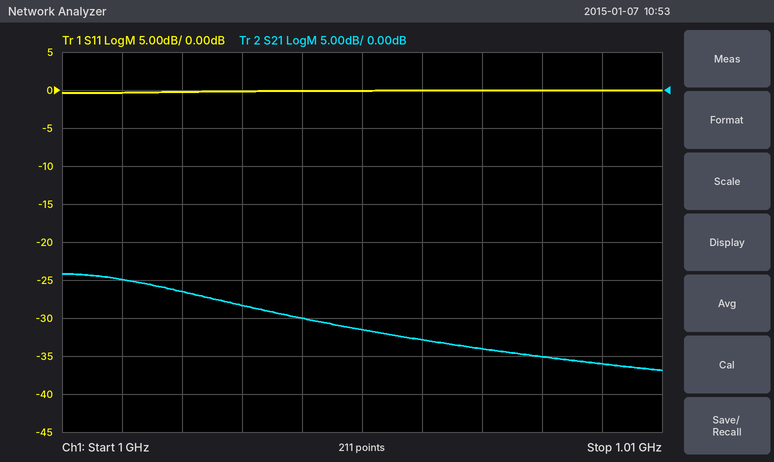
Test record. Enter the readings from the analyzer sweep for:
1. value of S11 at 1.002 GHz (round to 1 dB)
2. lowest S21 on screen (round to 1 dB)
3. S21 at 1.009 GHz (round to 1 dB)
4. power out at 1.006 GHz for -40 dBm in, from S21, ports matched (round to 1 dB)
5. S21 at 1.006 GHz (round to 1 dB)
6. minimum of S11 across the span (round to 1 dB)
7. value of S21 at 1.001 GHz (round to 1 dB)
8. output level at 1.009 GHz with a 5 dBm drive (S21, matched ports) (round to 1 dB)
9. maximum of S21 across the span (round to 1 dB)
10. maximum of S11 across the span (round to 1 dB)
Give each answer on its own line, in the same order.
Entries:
0 dB
-37 dB
-36 dB
-73 dBm
-33 dB
0 dB
-25 dB
-31 dBm
-24 dB
0 dB
